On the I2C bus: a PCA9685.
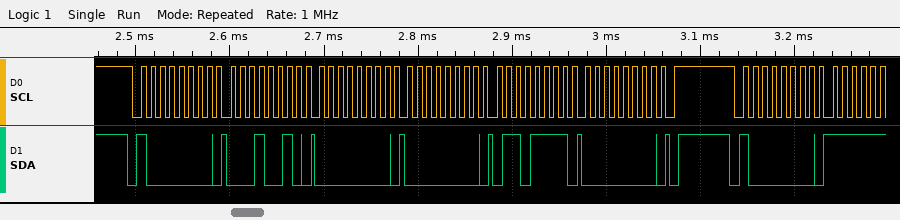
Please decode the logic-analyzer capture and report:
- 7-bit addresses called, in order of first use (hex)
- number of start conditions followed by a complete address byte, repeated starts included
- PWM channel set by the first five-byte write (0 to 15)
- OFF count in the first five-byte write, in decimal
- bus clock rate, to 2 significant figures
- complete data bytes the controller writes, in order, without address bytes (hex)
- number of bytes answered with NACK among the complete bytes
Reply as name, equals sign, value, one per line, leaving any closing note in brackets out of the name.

7-bit addresses called, in order of first use = 0x40
number of start conditions followed by a complete address byte, repeated starts included = 2
PWM channel set by the first five-byte write = 3
OFF count in the first five-byte write, in decimal = 111
bus clock rate, to 2 significant figures = 100 kHz
complete data bytes the controller writes, in order, without address bytes = 12 00 00 6F 00
number of bytes answered with NACK among the complete bytes = 0
